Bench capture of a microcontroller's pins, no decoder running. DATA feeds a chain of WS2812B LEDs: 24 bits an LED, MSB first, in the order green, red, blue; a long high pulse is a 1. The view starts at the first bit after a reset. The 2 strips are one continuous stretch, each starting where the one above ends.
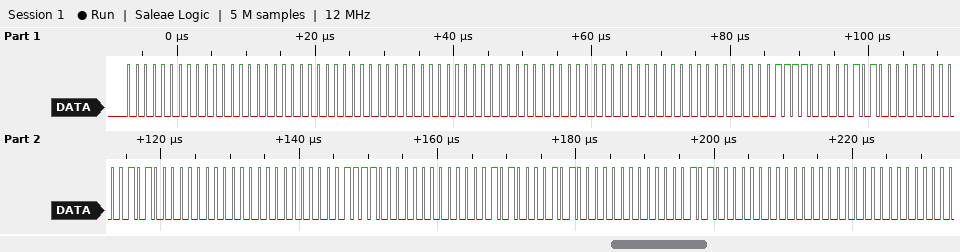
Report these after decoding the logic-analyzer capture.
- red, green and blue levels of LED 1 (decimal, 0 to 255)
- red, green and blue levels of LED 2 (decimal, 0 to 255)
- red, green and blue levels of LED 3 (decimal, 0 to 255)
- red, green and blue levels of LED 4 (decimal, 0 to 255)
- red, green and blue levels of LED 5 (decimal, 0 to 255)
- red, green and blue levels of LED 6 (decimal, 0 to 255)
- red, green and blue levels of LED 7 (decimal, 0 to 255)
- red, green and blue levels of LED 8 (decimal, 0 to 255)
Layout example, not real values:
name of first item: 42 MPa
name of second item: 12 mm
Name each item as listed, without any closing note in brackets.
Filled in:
red, green and blue levels of LED 1: 0, 0, 0
red, green and blue levels of LED 2: 0, 0, 0
red, green and blue levels of LED 3: 0, 0, 0
red, green and blue levels of LED 4: 10, 30, 0
red, green and blue levels of LED 5: 0, 40, 0
red, green and blue levels of LED 6: 0, 30, 10
red, green and blue levels of LED 7: 0, 20, 20
red, green and blue levels of LED 8: 0, 0, 0
